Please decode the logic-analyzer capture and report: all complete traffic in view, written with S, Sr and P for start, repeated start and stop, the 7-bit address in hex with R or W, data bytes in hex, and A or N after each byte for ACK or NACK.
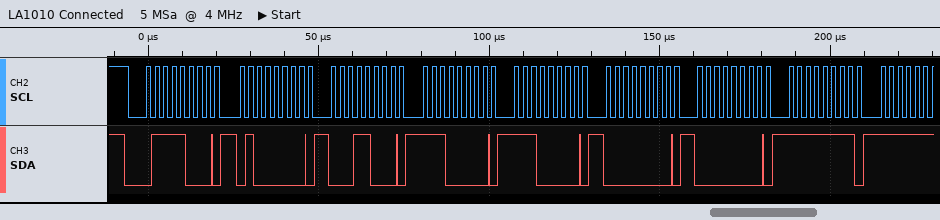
S 3CW A 40 A 18 A E0 A E0 A 00 A 00 A FF A
